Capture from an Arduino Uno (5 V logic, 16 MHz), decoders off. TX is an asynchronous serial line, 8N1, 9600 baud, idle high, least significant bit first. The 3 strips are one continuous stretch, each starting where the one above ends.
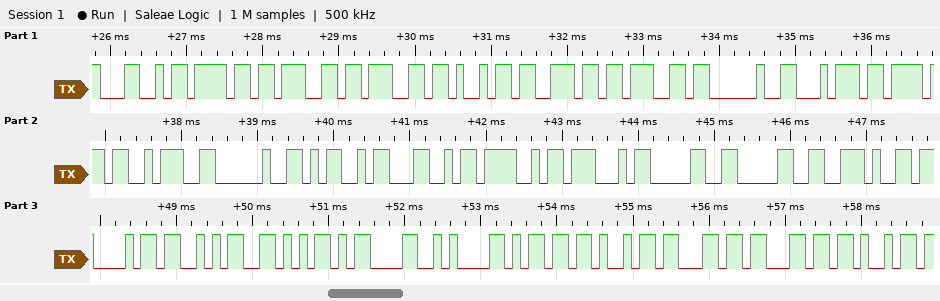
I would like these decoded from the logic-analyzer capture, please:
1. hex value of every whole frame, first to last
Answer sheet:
4C 6F 67 67 69 6E 67 20 74 6F 3A 20 4D 4C 4F 47 30 30 2E 43 53 56 0D 0A 6D 69 6C 6C 69
